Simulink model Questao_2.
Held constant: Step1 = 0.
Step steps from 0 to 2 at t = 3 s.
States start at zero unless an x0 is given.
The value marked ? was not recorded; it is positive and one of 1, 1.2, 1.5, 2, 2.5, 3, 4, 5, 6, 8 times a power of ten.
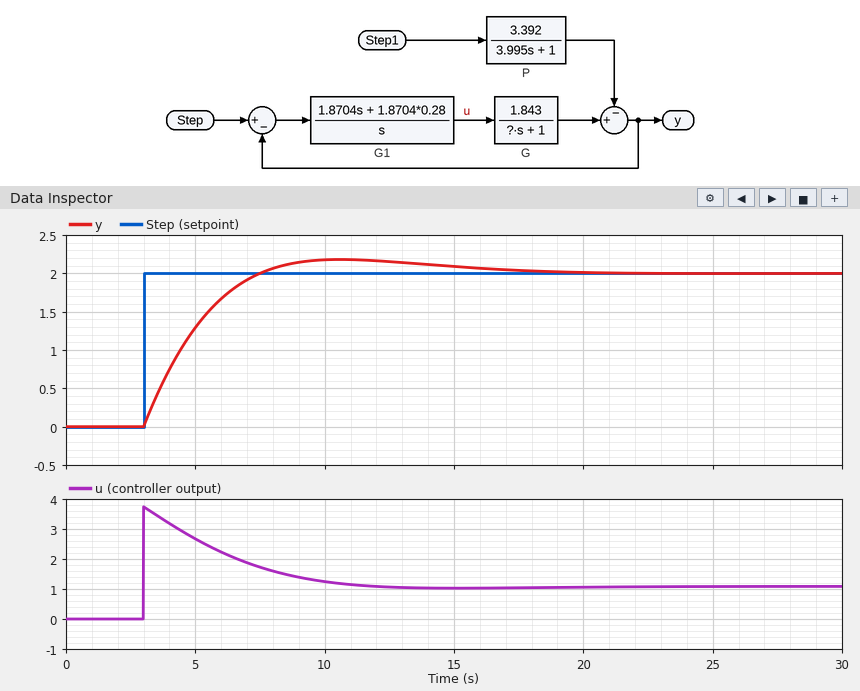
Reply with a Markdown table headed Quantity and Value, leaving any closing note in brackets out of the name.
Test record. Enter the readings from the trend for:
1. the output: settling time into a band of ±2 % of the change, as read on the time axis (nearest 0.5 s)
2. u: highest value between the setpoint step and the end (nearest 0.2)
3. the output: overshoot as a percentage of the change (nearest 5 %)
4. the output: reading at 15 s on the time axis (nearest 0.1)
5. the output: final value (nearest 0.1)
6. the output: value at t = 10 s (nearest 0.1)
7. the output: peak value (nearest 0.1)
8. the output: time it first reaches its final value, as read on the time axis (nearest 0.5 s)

| Quantity | Value |
|---|---|
| the output: settling time into a band of ±2 % of the change, as read on the time axis | 17.5 s |
| u: highest value between the setpoint step and the end | 3.8 |
| the output: overshoot as a percentage of the change | 10 % |
| the output: reading at 15 s on the time axis | 2.1 |
| the output: final value | 2.0 |
| the output: value at t = 10 s | 2.2 |
| the output: peak value | 2.2 |
| the output: time it first reaches its final value, as read on the time axis | 7.5 s |
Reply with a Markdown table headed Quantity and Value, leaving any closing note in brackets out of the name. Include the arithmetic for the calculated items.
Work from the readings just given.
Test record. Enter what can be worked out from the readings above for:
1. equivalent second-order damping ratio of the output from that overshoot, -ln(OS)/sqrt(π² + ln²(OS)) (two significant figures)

| Quantity | Value |
|---|---|
| equivalent second-order damping ratio of the output from that overshoot, -ln(OS)/sqrt(π² + ln²(OS)) | ln(0.1) = -2.303; 2.303 / sqrt(9.870 + 5.302) = 0.59 |
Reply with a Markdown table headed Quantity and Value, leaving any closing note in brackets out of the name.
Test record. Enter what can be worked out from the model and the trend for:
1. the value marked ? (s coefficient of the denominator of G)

| Quantity | Value |
|---|---|
| the value marked ? | 8 |
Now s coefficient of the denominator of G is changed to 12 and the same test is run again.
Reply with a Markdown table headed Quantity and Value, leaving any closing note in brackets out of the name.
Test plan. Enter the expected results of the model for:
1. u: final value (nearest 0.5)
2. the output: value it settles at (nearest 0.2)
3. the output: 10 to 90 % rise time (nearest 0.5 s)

| Quantity | Value |
|---|---|
| u: final value | 1.0 |
| the output: value it settles at | 2.0 |
| the output: 10 to 90 % rise time | 4.0 s |
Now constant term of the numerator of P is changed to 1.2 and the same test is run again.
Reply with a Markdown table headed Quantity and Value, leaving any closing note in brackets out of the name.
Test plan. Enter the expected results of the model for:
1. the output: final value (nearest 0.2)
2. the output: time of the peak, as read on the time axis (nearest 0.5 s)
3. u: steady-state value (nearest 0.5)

| Quantity | Value |
|---|---|
| the output: final value | 2.0 |
| the output: time of the peak, as read on the time axis | 10.5 s |
| u: steady-state value | 1.0 |
